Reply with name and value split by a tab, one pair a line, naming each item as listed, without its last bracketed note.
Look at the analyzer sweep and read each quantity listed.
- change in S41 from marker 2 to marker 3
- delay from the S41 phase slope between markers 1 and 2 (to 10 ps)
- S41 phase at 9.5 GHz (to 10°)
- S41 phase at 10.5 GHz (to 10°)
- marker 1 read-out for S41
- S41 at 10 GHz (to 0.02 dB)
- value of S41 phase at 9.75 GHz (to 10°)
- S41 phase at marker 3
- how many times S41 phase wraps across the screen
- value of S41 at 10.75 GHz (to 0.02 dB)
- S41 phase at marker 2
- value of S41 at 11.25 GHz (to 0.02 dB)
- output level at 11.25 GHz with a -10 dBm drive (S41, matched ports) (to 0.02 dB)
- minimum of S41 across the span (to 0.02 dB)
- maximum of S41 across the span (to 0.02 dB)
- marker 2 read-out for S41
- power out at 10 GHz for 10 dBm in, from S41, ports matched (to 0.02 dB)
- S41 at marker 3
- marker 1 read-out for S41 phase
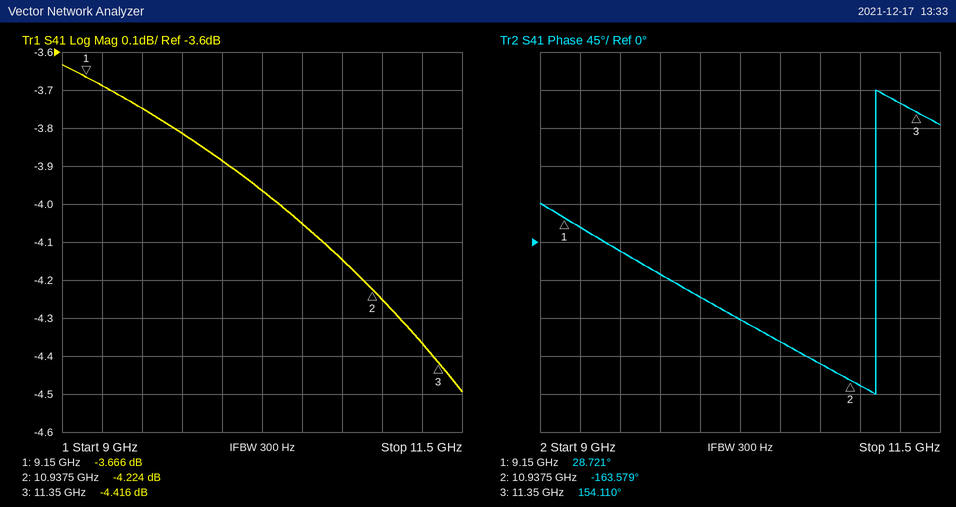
change in S41 from marker 2 to marker 3	-0.192 dB
delay from the S41 phase slope between markers 1 and 2	300 ps
S41 phase at 9.5 GHz	-10°
S41 phase at 10.5 GHz	-120°
marker 1 read-out for S41	-3.666 dB
S41 at 10 GHz	-3.88 dB
value of S41 phase at 9.75 GHz	-40°
S41 phase at marker 3	154.110°
how many times S41 phase wraps across the screen	1
value of S41 at 10.75 GHz	-4.14 dB
S41 phase at marker 2	-163.579°
value of S41 at 11.25 GHz	-4.36 dB
output level at 11.25 GHz with a -10 dBm drive (S41, matched ports)	-14.36 dBm
minimum of S41 across the span	-4.50 dB
maximum of S41 across the span	-3.64 dB
marker 2 read-out for S41	-4.224 dB
power out at 10 GHz for 10 dBm in, from S41, ports matched	6.12 dBm
S41 at marker 3	-4.416 dB
marker 1 read-out for S41 phase	28.721°
